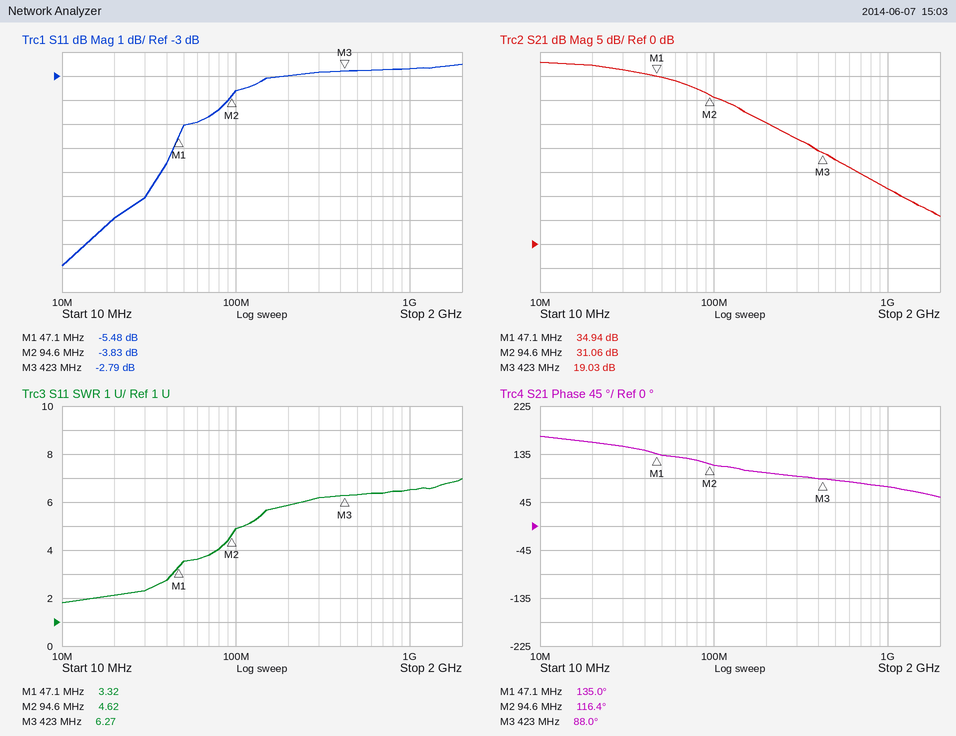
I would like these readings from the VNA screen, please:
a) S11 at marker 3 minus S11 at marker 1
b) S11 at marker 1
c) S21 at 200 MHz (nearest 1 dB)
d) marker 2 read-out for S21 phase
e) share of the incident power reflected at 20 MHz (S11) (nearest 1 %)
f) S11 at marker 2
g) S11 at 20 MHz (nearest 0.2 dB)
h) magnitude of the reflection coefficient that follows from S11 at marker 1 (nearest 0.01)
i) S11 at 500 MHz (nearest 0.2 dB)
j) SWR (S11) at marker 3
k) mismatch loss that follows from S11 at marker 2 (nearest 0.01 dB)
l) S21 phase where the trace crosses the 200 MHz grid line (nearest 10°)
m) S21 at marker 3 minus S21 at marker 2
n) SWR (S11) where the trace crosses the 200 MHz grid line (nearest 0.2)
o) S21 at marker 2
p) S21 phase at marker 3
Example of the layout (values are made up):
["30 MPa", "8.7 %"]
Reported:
["2.69 dB", "-5.48 dB", "25 dB", "116.4°", "13 %", "-3.83 dB", "-9.0 dB", "0.53", "-2.8 dB", "6.27", "2.32 dB", "100°", "-12.03 dB", "5.8", "31.06 dB", "88.0°"]
